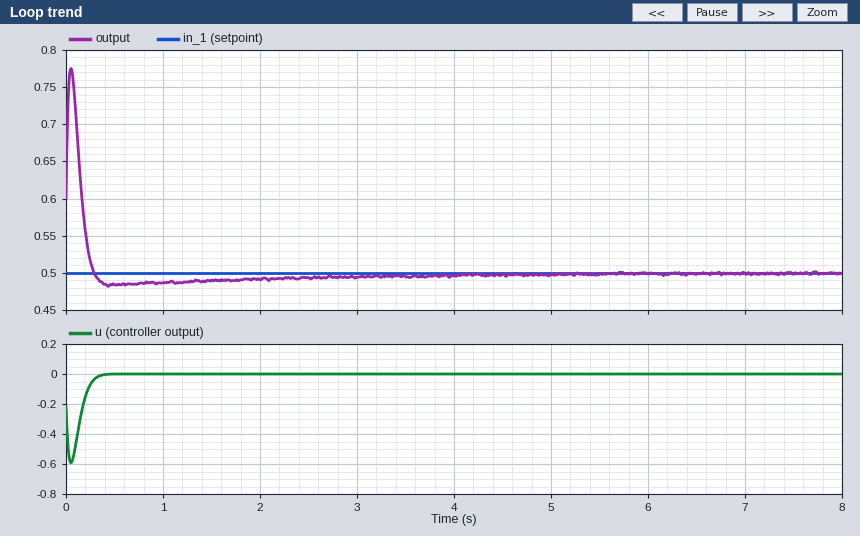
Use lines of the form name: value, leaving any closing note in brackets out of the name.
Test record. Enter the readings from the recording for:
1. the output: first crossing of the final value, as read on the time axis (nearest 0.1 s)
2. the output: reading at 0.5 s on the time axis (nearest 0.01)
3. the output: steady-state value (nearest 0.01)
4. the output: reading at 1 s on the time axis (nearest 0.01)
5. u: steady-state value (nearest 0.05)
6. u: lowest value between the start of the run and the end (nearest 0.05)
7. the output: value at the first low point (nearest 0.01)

the output: first crossing of the final value, as read on the time axis: 0.3 s
the output: reading at 0.5 s on the time axis: 0.48
the output: steady-state value: 0.50
the output: reading at 1 s on the time axis: 0.49
u: steady-state value: 0.00
u: lowest value between the start of the run and the end: -0.60
the output: value at the first low point: 0.48
